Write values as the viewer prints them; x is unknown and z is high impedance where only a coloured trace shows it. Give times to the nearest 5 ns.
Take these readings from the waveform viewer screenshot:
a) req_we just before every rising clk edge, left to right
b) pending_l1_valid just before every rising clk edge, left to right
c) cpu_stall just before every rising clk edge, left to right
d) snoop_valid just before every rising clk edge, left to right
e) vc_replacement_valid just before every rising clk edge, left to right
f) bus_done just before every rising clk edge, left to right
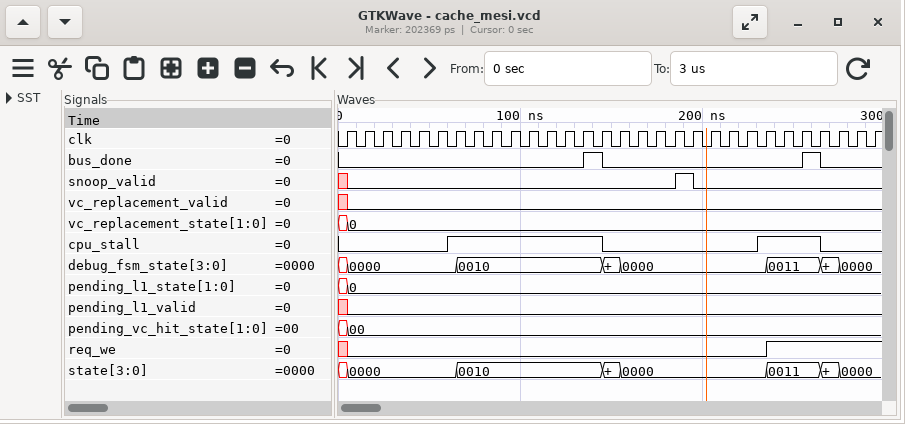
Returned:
x 0 0 0 0 0 0 0 0 0 0 0 0 0 0 0 0 0 0 0 0 0 0 0 1 1 1 1 1 1
x 0 0 0 0 0 0 0 0 0 0 0 0 0 0 0 0 0 0 0 0 0 0 0 0 0 0 0 0 0
0 0 0 0 0 0 1 1 1 1 1 1 1 1 1 0 0 0 0 0 0 0 0 1 1 1 1 0 0 0
x 0 0 0 0 0 0 0 0 0 0 0 0 0 0 0 0 0 0 1 0 0 0 0 0 0 0 0 0 0
x 0 0 0 0 0 0 0 0 0 0 0 0 0 0 0 0 0 0 0 0 0 0 0 0 0 0 0 0 0
0 0 0 0 0 0 0 0 0 0 0 0 0 0 1 0 0 0 0 0 0 0 0 0 0 0 1 0 0 0
